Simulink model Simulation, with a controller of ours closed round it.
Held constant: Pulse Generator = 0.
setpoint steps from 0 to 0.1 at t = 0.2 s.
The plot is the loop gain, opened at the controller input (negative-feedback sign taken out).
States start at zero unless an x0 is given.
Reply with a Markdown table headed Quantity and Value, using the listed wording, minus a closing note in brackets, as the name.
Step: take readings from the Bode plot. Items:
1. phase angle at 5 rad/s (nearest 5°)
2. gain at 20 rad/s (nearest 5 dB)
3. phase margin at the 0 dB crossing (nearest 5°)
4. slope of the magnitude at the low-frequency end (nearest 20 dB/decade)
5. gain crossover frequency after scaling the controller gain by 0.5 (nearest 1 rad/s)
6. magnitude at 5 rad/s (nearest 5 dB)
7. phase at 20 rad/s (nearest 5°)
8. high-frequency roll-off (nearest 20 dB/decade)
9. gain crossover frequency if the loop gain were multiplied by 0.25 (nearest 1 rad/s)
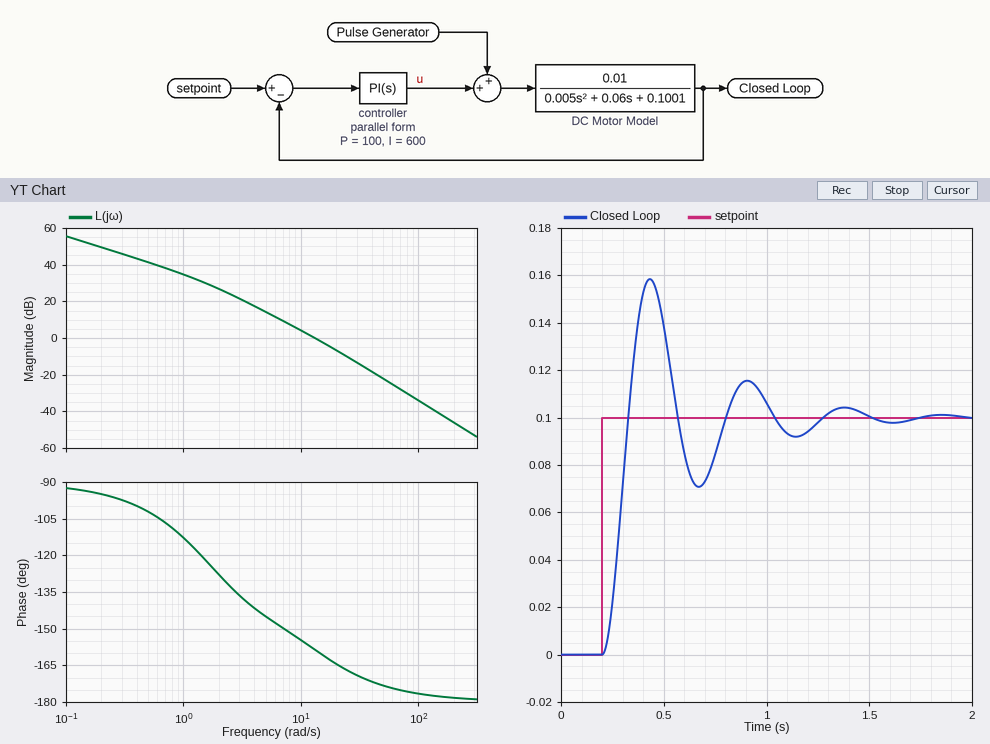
| Quantity | Value |
|---|---|
| phase angle at 5 rad/s | -145° |
| gain at 20 rad/s | -5 dB |
| phase margin at the 0 dB crossing | 20° |
| slope of the magnitude at the low-frequency end | -20 dB/decade |
| gain crossover frequency after scaling the controller gain by 0.5 | 9 rad/s |
| magnitude at 5 rad/s | 15 dB |
| phase at 20 rad/s | -165° |
| high-frequency roll-off | -40 dB/decade |
| gain crossover frequency if the loop gain were multiplied by 0.25 | 6 rad/s |
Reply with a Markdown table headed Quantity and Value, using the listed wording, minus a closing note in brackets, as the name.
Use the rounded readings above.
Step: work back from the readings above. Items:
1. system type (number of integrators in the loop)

| Quantity | Value |
|---|---|
| system type | 1 |
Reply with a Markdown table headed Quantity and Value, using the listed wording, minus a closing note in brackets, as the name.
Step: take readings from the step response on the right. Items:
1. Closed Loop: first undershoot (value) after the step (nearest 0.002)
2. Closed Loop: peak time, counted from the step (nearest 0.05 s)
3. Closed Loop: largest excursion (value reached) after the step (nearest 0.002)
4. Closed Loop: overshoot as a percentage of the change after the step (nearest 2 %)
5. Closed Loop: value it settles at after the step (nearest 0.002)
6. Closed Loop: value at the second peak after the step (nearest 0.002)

| Quantity | Value |
|---|---|
| Closed Loop: first undershoot (value) after the step | 0.070 |
| Closed Loop: peak time, counted from the step | 0.25 s |
| Closed Loop: largest excursion (value reached) after the step | 0.158 |
| Closed Loop: overshoot as a percentage of the change after the step | 58 % |
| Closed Loop: value it settles at after the step | 0.100 |
| Closed Loop: value at the second peak after the step | 0.116 |
